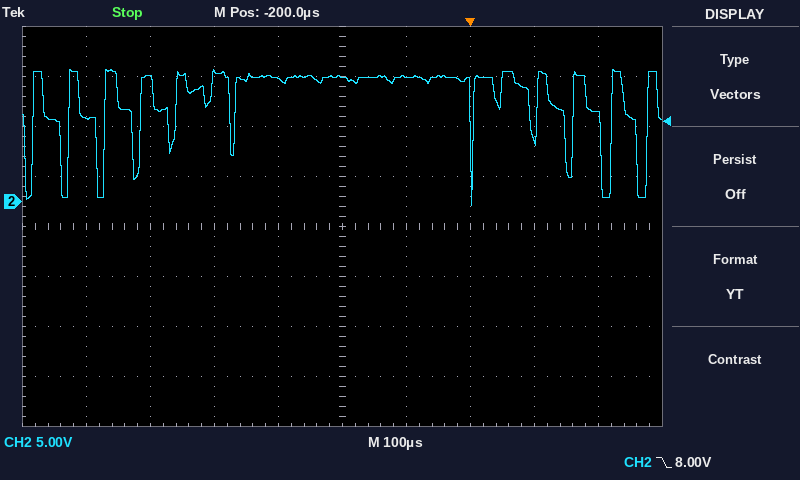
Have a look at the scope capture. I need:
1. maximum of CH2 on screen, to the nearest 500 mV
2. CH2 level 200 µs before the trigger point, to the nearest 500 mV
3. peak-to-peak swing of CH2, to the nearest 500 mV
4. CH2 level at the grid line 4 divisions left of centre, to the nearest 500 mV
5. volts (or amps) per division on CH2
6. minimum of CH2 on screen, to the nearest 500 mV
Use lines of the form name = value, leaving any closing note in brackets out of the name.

maximum of CH2 on screen, to the nearest 500 mV = 13.0 V
CH2 level 200 µs before the trigger point, to the nearest 500 mV = 12.5 V
peak-to-peak swing of CH2, to the nearest 500 mV = 13.5 V
CH2 level at the grid line 4 divisions left of centre, to the nearest 500 mV = 8.5 V
volts (or amps) per division on CH2 = 5 V
minimum of CH2 on screen, to the nearest 500 mV = -500 mV
